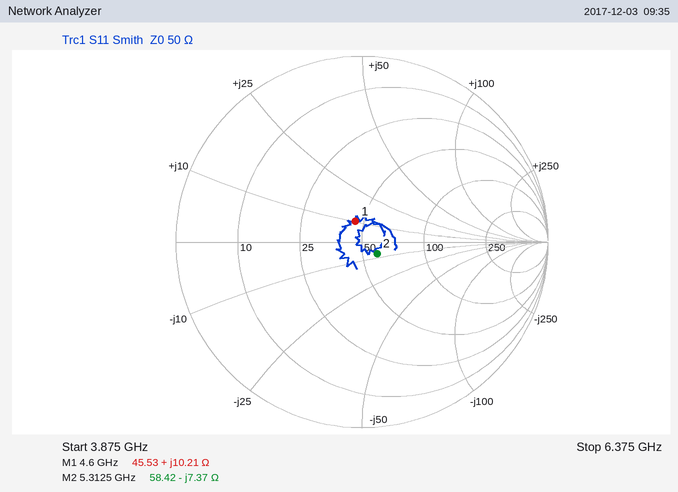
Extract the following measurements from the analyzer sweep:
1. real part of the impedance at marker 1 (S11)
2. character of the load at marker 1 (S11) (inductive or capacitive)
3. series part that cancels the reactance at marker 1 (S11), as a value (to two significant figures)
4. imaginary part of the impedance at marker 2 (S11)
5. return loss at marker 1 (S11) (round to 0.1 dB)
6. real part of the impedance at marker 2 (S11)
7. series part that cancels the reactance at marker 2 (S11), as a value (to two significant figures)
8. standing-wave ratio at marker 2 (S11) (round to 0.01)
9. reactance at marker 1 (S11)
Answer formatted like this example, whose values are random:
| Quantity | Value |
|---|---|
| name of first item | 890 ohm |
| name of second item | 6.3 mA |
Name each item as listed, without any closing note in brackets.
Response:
| Quantity | Value |
|---|---|
| real part of the impedance at marker 1 | 45.53 Ω |
| character of the load at marker 1 (S11) | inductive |
| series part that cancels the reactance at marker 1 (S11), as a value | 3.4 pF |
| imaginary part of the impedance at marker 2 | -7.37 Ω |
| return loss at marker 1 (S11) | 18.7 dB |
| real part of the impedance at marker 2 | 58.42 Ω |
| series part that cancels the reactance at marker 2 (S11), as a value | 220 pH |
| standing-wave ratio at marker 2 (S11) | 1.23 |
| reactance at marker 1 | +10.21 Ω |
